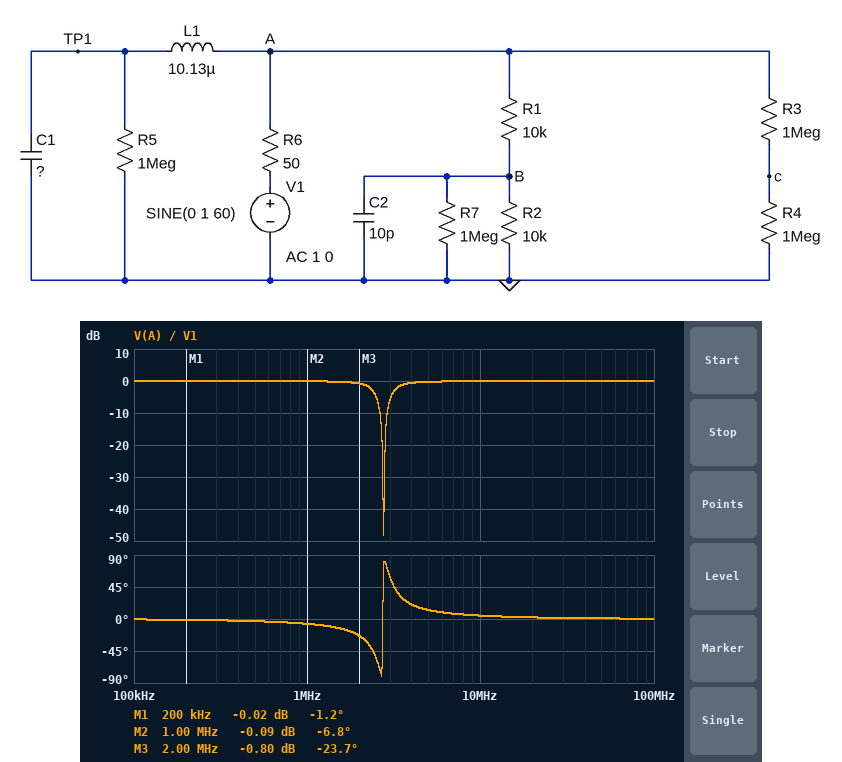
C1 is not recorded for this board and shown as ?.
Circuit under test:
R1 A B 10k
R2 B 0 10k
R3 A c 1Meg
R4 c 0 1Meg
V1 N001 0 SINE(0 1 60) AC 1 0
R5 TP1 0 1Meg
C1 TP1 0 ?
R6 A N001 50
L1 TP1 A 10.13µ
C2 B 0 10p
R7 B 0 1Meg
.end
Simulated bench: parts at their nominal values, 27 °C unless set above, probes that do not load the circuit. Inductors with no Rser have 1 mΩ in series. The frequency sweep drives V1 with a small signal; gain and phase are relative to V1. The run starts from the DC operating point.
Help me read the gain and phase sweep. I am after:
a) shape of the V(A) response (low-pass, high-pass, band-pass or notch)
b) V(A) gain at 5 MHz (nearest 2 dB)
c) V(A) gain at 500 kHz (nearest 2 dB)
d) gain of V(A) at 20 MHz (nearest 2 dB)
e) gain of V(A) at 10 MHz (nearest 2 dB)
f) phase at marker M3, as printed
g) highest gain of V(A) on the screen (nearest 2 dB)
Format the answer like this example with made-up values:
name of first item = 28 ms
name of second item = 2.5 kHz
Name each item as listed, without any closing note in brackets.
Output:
shape of the V(A) response = notch
V(A) gain at 5 MHz = 0 dB
V(A) gain at 500 kHz = 0 dB
gain of V(A) at 20 MHz = 0 dB
gain of V(A) at 10 MHz = 0 dB
phase at marker M3, as printed = -23.7 deg
highest gain of V(A) on the screen = 0 dB
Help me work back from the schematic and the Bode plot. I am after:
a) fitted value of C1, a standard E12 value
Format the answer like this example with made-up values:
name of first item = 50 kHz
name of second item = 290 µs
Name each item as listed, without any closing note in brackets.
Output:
fitted value of C1, a standard E12 value = 330 pF
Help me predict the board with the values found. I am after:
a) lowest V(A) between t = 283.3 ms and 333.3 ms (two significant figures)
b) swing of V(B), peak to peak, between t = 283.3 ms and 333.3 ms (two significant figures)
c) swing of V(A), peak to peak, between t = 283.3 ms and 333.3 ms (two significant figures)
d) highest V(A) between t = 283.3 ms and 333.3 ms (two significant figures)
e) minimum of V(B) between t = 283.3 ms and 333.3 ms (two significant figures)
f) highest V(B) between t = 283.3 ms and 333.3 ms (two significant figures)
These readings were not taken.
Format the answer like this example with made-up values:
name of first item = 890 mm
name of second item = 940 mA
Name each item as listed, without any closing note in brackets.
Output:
lowest V(A) between t = 283.3 ms and 333.3 ms = -1.0 V
swing of V(B), peak to peak, between t = 283.3 ms and 333.3 ms = 990 mV
swing of V(A), peak to peak, between t = 283.3 ms and 333.3 ms = 2.0 V
highest V(A) between t = 283.3 ms and 333.3 ms = 1.0 V
minimum of V(B) between t = 283.3 ms and 333.3 ms = -500 mV
highest V(B) between t = 283.3 ms and 333.3 ms = 500 mV
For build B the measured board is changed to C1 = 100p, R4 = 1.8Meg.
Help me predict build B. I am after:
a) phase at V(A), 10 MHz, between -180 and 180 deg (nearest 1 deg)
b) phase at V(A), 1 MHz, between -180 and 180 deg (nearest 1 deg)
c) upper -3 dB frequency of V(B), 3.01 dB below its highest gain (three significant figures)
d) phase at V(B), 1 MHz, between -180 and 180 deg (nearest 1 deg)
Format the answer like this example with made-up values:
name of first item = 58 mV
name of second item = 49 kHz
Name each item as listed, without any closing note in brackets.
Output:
phase at V(A), 10 MHz, between -180 and 180 deg = 6 deg
phase at V(A), 1 MHz, between -180 and 180 deg = -2 deg
upper -3 dB frequency of V(B), 3.01 dB below its highest gain = 3.11 MHz
phase at V(B), 1 MHz, between -180 and 180 deg = -19 deg
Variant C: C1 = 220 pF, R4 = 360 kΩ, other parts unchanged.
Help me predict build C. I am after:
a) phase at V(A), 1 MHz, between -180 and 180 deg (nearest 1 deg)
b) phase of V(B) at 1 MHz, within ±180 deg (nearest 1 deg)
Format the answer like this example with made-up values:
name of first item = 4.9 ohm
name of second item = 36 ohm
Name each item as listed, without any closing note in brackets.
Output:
phase at V(A), 1 MHz, between -180 and 180 deg = -4 deg
phase of V(B) at 1 MHz, within ±180 deg = -22 deg
